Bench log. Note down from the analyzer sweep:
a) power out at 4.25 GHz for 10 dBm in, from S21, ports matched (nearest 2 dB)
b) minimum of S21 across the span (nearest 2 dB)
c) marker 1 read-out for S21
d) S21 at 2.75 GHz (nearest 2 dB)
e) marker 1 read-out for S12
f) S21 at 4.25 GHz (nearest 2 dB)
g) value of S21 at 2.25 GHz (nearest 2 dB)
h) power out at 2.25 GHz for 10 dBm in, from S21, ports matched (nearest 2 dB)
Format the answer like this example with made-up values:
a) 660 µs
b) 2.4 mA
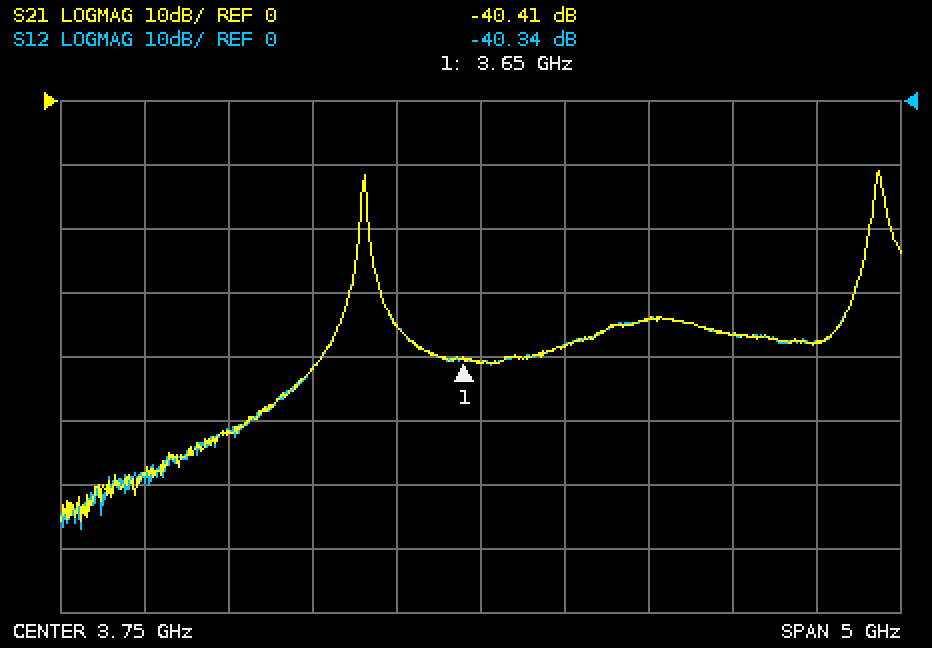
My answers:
a) -28 dBm
b) -66 dB
c) -40.41 dB
d) -42 dB
e) -40.34 dB
f) -38 dB
g) -52 dB
h) -42 dBm
